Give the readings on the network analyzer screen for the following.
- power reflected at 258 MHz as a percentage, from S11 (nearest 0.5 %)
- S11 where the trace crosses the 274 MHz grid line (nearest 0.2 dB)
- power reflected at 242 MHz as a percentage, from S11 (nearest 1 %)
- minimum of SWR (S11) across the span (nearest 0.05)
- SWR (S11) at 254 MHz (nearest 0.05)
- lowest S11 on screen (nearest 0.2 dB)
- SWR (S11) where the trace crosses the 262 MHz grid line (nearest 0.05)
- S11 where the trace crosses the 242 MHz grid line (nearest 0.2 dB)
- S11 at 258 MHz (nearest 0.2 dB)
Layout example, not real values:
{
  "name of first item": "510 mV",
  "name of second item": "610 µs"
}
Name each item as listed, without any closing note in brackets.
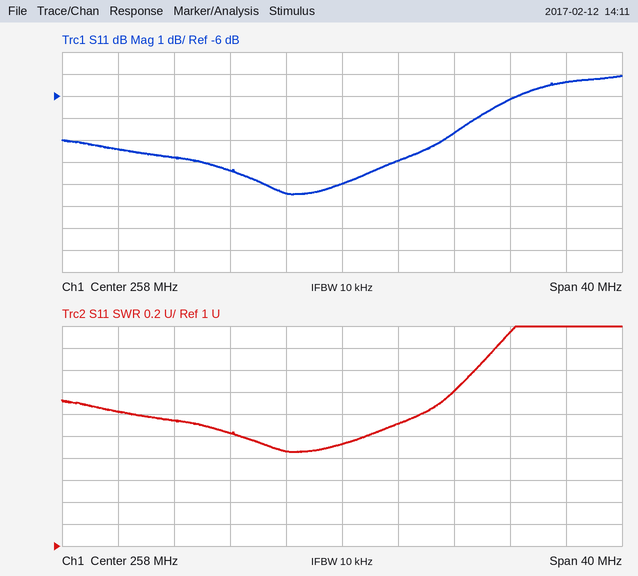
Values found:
{
  "power reflected at 258 MHz as a percentage, from S11": "10.0 %",
  "S11 where the trace crosses the 274 MHz grid line": "-5.4 dB",
  "power reflected at 242 MHz as a percentage, from S11": "14 %",
  "minimum of SWR (S11) across the span": "1.85",
  "SWR (S11) at 254 MHz": "1.85",
  "lowest S11 on screen": "-10.4 dB",
  "SWR (S11) where the trace crosses the 262 MHz grid line": "2.10",
  "S11 where the trace crosses the 242 MHz grid line": "-8.4 dB",
  "S11 at 258 MHz": "-10.0 dB"
}
